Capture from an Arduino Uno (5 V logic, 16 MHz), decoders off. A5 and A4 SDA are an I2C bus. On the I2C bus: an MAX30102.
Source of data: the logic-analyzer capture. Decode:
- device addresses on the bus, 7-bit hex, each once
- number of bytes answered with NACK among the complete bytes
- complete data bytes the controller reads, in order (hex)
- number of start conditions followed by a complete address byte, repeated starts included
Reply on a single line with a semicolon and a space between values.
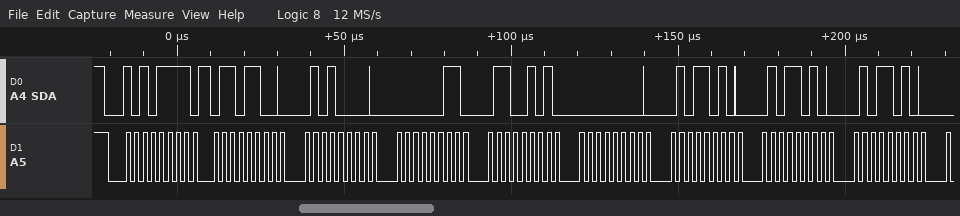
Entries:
0x57; 0; 6C 50 03 65 00 5A 5A 5A; 1
